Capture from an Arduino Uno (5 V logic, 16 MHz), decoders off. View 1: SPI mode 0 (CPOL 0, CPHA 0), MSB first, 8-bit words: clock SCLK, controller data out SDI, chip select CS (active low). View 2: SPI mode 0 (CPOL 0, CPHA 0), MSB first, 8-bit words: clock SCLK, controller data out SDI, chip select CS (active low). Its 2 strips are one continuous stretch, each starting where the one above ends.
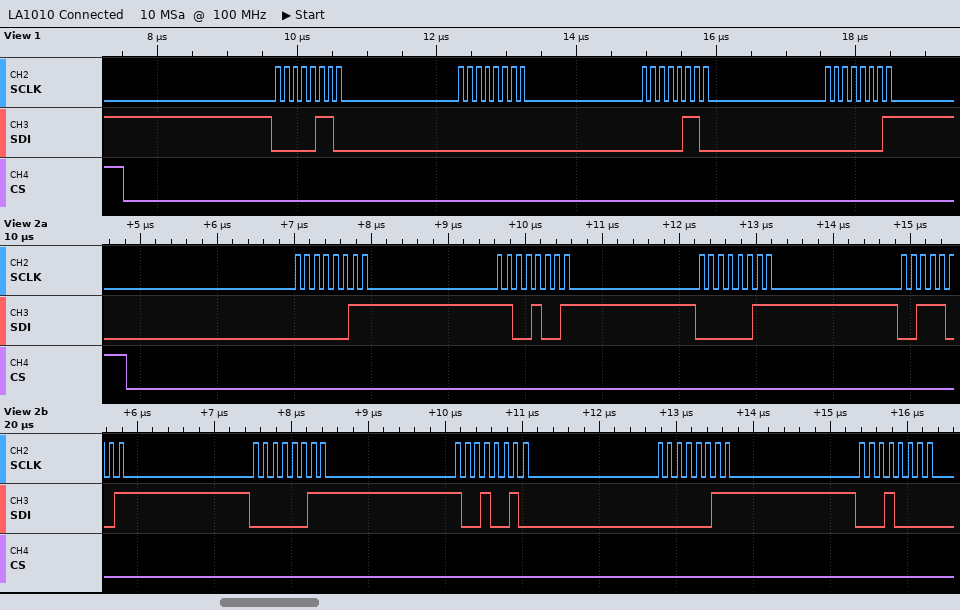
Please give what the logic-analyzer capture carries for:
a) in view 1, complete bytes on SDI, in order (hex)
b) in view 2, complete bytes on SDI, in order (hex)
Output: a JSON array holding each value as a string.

["06 00 06 01", "03 C9 03 39 03 92 03 10"]
